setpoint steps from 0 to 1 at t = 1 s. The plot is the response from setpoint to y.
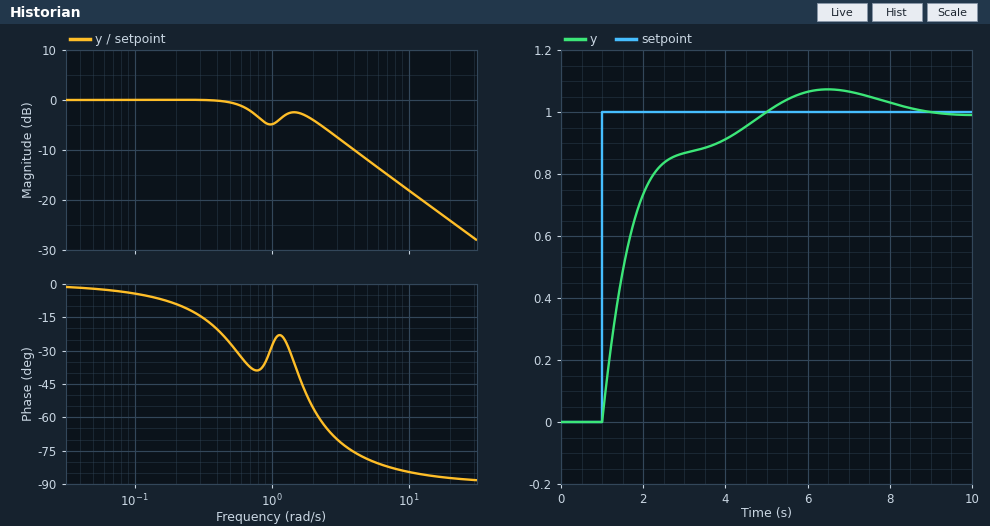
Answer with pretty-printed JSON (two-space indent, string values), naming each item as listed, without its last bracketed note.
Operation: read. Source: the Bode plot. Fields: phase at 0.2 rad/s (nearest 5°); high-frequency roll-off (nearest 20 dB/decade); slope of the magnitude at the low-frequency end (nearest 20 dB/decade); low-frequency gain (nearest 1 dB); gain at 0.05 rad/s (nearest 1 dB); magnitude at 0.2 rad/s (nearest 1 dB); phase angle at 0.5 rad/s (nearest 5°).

{
  "phase at 0.2 rad/s": "-10°",
  "high-frequency roll-off": "-20 dB/decade",
  "slope of the magnitude at the low-frequency end": "0 dB/decade",
  "low-frequency gain": "0 dB",
  "gain at 0.05 rad/s": "0 dB",
  "magnitude at 0.2 rad/s": "0 dB",
  "phase angle at 0.5 rad/s": "-25°"
}
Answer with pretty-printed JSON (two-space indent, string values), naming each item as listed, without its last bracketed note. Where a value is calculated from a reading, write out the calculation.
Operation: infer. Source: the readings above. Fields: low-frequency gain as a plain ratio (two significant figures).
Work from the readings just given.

{
  "low-frequency gain as a plain ratio": "10^(0 / 20) = 1.0"
}
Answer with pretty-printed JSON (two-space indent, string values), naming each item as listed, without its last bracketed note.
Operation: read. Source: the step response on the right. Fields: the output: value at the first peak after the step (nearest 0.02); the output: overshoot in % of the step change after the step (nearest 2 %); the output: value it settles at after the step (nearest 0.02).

{
  "the output: value at the first peak after the step": "1.08",
  "the output: overshoot in % of the step change after the step": "8 %",
  "the output: value it settles at after the step": "1.00"
}
